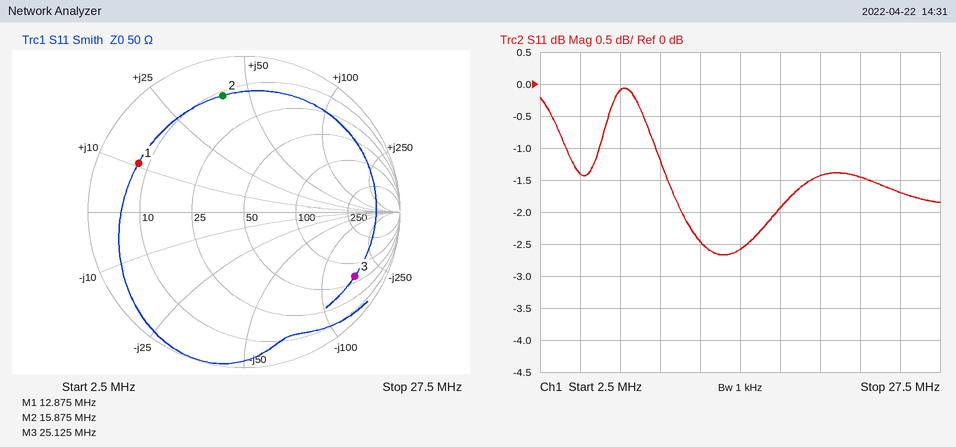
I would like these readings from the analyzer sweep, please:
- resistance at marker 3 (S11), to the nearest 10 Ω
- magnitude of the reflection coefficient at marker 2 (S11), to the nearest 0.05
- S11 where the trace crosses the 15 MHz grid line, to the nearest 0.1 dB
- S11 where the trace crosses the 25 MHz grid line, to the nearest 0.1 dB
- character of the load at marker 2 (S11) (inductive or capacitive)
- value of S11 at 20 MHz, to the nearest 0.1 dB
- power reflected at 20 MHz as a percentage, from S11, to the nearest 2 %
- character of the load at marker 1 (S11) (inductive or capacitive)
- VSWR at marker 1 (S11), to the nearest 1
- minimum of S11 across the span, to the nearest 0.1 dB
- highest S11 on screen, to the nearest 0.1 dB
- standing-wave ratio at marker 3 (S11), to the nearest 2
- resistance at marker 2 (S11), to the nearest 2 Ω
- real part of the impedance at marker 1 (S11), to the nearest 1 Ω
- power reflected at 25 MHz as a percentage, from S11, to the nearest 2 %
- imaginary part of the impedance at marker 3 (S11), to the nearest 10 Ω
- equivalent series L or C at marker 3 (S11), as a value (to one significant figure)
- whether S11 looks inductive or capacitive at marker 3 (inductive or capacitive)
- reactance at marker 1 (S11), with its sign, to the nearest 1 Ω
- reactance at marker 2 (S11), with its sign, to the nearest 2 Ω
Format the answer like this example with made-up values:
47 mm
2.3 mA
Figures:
60 Ω
0.75
-2.6 dB
-1.7 dB
inductive
-1.4 dB
72 %
inductive
7
-2.7 dB
-0.1 dB
10
12 Ω
8 Ω
68 %
-160 Ω
40 pF
capacitive
+11 Ω
+40 Ω
